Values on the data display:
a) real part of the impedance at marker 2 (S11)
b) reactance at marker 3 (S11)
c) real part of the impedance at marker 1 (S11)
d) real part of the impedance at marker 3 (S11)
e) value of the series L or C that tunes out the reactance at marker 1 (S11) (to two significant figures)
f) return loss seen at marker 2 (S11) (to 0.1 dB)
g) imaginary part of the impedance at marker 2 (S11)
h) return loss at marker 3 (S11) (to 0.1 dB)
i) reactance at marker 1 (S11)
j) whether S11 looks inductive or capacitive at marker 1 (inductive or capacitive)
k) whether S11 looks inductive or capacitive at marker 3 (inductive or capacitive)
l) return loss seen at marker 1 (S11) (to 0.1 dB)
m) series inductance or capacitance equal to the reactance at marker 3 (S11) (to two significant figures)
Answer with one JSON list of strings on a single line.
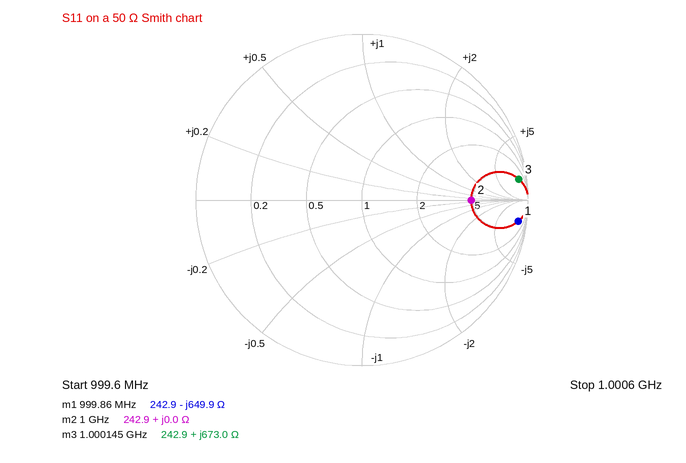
["242.9 Ω", "+673.0 Ω", "242.9 Ω", "242.9 Ω", "100 nH", "3.6 dB", "+0.0 Ω", "0.4 dB", "-649.9 Ω", "capacitive", "inductive", "0.4 dB", "110 nH"]
